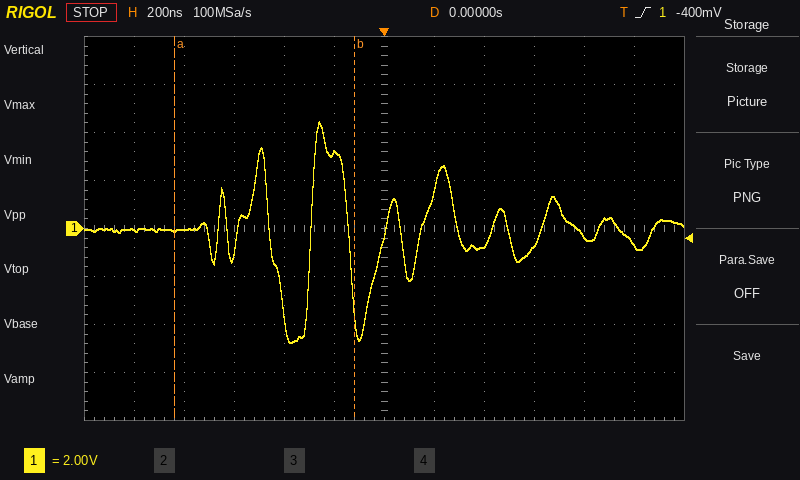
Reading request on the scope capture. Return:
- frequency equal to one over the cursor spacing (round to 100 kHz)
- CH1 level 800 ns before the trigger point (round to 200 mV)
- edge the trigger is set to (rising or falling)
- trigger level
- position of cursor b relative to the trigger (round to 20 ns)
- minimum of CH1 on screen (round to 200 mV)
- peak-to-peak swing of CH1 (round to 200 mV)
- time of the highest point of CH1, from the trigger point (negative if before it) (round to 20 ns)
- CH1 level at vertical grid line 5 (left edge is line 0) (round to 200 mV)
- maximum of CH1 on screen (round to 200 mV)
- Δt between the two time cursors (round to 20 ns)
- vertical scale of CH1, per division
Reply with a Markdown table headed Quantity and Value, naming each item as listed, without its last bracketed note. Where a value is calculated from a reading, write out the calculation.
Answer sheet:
| Quantity | Value |
|---|---|
| frequency equal to one over the cursor spacing | 1 / 720 ns ≈ 1.4 MHz |
| CH1 level 800 ns before the trigger point | 0.0 V |
| edge the trigger is set to | rising |
| trigger level | -400 mV |
| position of cursor b relative to the trigger | -120 ns |
| minimum of CH1 on screen | -4.8 V |
| peak-to-peak swing of CH1 | 4.4 V − (-4.8 V) = 9.2 V |
| time of the highest point of CH1, from the trigger point (negative if before it) | -260 ns |
| CH1 level at vertical grid line 5 (left edge is line 0) | 3.2 V |
| maximum of CH1 on screen | 4.4 V |
| Δt between the two time cursors | 720 ns |
| vertical scale of CH1, per division | 2 V |
